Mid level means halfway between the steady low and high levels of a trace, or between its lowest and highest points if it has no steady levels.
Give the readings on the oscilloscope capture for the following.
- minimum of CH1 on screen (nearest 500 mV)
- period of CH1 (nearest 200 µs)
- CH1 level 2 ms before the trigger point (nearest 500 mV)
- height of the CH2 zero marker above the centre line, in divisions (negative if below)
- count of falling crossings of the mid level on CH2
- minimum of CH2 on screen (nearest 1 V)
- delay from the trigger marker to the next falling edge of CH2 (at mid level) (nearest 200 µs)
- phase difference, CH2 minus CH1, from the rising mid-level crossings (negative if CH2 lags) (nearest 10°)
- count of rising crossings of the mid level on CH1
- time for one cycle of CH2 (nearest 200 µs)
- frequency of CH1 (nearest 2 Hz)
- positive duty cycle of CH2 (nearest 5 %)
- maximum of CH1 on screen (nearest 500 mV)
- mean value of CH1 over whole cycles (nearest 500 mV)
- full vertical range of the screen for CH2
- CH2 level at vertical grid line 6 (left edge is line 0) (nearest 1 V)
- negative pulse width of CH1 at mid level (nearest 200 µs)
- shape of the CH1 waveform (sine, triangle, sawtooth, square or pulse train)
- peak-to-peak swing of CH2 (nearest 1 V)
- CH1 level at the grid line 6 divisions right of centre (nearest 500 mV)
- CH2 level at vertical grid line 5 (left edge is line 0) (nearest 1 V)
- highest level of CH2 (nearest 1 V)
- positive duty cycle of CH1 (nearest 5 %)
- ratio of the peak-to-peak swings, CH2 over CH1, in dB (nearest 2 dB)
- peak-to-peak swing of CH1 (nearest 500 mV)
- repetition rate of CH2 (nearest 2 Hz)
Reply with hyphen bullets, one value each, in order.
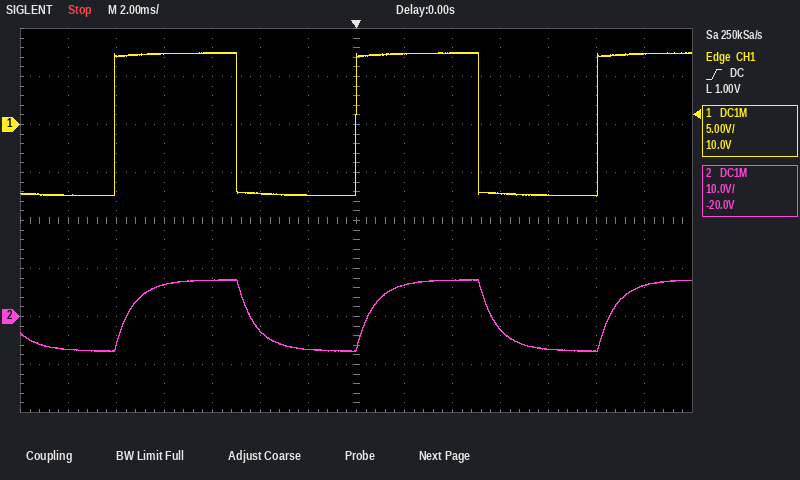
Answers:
- -7.5 V
- 10.0 ms
- -7.5 V
- -2.0 div
- 2
- -7 V
- 5.6 ms
- -20°
- 3
- 10.0 ms
- 100 Hz
- 50 %
- 7.5 V
- 0.0 V
- 80 V
- -7 V
- 5.0 ms
- square
- 15 V
- 7.5 V
- -3 V
- 8 V
- 50 %
- 0 dB
- 15.0 V
- 100 Hz
